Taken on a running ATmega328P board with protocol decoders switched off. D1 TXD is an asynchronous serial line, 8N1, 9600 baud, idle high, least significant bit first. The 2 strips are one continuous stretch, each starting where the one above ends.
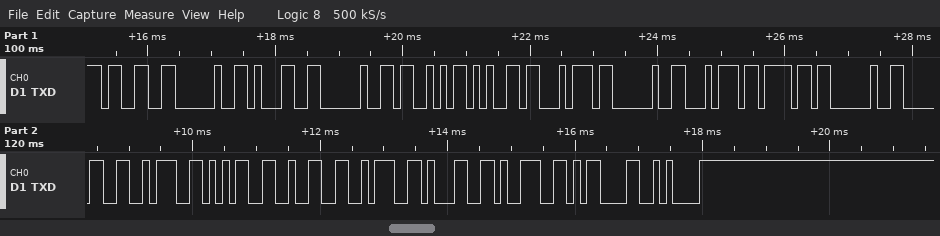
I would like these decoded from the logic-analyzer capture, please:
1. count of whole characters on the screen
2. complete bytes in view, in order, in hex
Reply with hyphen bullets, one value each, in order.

- 20
- 0x33 0x20 0x31 0x20 0x53 0x65 0x74 0x20 0x74 0x6F 0x20 0x30 0x3A 0x35 0x32 0x3A 0x31 0x39 0x0D 0x0A
